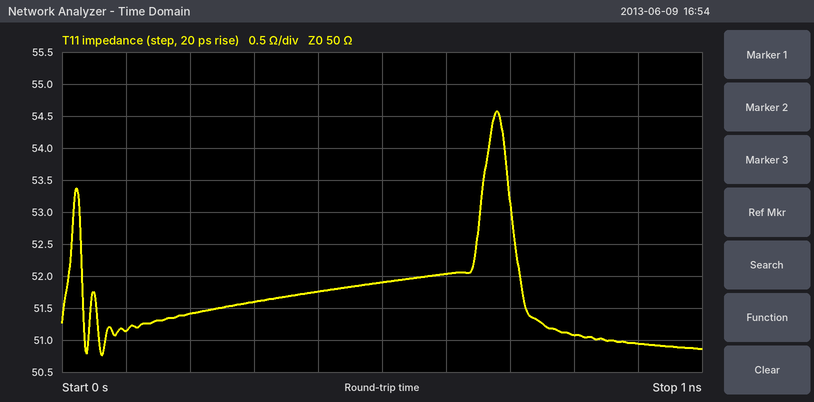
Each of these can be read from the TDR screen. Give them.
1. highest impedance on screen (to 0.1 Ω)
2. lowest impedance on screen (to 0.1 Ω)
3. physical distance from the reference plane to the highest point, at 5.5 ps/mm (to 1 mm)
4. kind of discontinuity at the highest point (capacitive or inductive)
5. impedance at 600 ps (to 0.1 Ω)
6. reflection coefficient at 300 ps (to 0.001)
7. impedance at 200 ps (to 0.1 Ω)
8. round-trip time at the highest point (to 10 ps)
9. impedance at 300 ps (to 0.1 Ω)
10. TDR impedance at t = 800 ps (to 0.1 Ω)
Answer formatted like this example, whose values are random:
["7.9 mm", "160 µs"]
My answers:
["54.6 Ω", "50.8 Ω", "62 mm", "inductive", "52.0 Ω", "+0.016", "51.4 Ω", "680 ps", "51.6 Ω", "51.1 Ω"]
